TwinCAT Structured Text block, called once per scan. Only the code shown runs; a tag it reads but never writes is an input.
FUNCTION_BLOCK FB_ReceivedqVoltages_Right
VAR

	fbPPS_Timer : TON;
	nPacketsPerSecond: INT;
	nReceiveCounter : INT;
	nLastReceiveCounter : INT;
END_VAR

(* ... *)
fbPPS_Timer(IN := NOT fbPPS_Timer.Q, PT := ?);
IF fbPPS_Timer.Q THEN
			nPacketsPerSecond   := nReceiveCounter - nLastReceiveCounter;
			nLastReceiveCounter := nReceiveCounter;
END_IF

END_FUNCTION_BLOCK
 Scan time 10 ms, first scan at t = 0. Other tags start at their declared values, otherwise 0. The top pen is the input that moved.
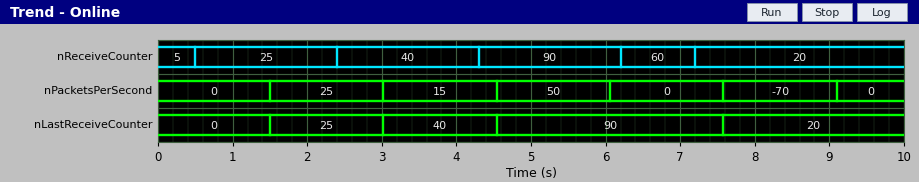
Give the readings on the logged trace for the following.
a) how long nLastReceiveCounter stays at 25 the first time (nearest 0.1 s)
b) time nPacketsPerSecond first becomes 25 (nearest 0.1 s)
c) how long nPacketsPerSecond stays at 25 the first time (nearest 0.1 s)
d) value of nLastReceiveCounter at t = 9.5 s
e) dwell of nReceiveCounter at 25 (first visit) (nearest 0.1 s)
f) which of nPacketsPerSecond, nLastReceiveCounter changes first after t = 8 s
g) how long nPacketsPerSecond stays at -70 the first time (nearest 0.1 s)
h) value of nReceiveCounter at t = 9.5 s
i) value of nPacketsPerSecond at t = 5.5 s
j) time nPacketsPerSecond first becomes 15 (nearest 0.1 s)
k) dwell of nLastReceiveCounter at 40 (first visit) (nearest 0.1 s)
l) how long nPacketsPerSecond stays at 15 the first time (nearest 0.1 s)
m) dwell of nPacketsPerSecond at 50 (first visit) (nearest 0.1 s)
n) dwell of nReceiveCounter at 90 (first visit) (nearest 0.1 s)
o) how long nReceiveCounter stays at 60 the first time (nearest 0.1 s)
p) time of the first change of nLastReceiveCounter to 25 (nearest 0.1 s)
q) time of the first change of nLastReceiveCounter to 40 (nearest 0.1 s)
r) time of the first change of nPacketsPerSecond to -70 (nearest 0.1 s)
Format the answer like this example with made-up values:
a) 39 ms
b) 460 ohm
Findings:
a) 1.5 s
b) 1.5 s
c) 1.5 s
d) 20
e) 1.9 s
f) nPacketsPerSecond
g) 1.5 s
h) 20
i) 50
j) 3.0 s
k) 1.5 s
l) 1.5 s
m) 1.5 s
n) 1.9 s
o) 1.0 s
p) 1.5 s
q) 3.0 s
r) 7.6 s
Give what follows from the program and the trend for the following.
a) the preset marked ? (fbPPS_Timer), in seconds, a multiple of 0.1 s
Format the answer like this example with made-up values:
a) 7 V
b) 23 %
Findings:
a) 1.5 s
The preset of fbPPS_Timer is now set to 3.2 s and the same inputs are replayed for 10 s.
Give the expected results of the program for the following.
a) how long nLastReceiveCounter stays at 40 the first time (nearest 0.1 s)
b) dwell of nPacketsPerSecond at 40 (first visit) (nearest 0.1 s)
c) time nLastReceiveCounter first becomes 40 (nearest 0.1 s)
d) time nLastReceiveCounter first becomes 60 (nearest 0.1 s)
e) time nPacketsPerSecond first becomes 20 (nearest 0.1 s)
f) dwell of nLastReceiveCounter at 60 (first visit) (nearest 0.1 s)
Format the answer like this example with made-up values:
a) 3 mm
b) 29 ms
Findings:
a) 3.2 s
b) 3.2 s
c) 3.2 s
d) 6.4 s
e) 6.4 s
f) 3.2 s
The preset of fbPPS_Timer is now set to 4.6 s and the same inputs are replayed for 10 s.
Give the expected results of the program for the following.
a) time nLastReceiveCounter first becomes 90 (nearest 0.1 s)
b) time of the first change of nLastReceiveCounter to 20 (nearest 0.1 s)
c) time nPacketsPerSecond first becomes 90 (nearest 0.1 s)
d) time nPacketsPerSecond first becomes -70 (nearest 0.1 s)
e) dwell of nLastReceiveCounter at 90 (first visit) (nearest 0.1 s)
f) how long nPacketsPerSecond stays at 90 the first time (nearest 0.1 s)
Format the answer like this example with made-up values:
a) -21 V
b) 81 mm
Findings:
a) 4.6 s
b) 9.2 s
c) 4.6 s
d) 9.2 s
e) 4.6 s
f) 4.6 s
